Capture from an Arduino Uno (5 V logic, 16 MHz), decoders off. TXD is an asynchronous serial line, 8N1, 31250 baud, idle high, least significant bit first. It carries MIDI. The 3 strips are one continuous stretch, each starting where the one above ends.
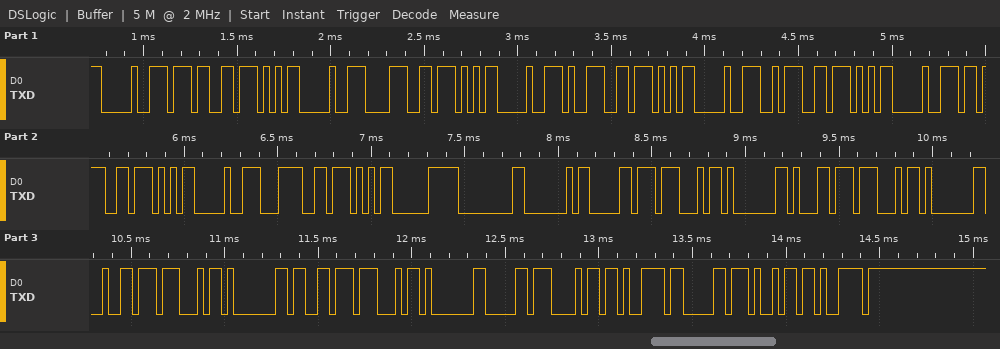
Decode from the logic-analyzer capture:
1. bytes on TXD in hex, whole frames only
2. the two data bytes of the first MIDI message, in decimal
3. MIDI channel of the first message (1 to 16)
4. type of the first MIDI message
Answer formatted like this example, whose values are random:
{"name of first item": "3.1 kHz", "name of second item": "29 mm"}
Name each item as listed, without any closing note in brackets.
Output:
{"bytes on TXD in hex, whole frames only": "90 37 57 90 38 57 90 39 57 90 3A 57 90 3B 57 90 3C 57 E0 00 40 B0 47 01 B1 47 01 B2 47 01 B3 47 01 B0 68 79 B0 69 79", "the two data bytes of the first MIDI message, in decimal": "55, 87", "MIDI channel of the first message": "1", "type of the first MIDI message": "Note On"}
